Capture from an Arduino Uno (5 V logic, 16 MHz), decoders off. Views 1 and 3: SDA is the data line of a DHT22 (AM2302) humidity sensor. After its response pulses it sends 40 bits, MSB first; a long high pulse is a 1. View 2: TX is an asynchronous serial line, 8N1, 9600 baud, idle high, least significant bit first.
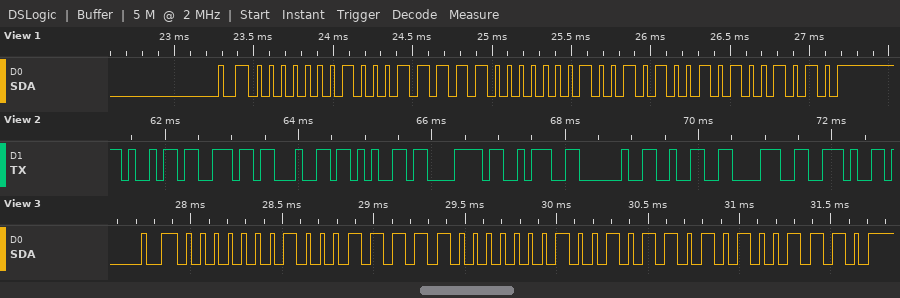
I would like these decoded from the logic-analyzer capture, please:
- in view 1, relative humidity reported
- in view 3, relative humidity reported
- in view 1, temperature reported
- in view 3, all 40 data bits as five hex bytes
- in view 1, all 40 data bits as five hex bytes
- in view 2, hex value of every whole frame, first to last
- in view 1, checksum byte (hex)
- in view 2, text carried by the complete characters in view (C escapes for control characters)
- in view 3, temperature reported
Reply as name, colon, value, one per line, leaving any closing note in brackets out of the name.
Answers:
in view 1, relative humidity reported: 28.7 %
in view 3, relative humidity reported: 28.7 %
in view 1, temperature reported: 29.7 °C
in view 3, all 40 data bits as five hex bytes: 01 1F 01 2D 4E
in view 1, all 40 data bits as five hex bytes: 01 1F 01 29 4A
in view 2, hex value of every whole frame, first to last: 69 6E 64 65 78 3A 20 32 38 2E
in view 1, checksum byte: 0x4A
in view 2, text carried by the complete characters in view: "index: 28."
in view 3, temperature reported: 30.1 °C
